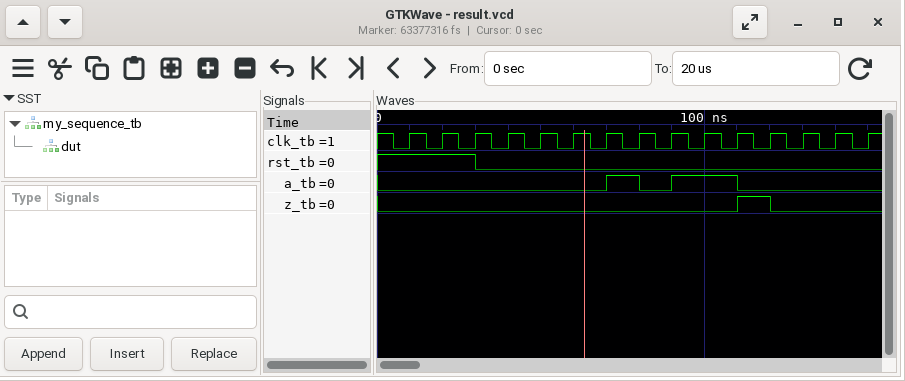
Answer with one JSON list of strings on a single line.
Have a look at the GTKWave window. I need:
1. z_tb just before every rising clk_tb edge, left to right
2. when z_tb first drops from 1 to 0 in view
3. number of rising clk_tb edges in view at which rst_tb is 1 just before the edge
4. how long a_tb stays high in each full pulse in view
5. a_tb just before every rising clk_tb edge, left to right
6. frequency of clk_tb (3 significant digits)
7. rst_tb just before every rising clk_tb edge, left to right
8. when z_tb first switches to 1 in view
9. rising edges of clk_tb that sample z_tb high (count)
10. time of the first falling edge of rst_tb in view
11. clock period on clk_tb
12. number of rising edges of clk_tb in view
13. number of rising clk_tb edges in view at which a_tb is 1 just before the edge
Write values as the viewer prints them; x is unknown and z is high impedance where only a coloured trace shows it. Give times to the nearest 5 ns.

["0 0 0 0 0 0 0 0 0 0 0 1 0 0 0", "120 ns", "3", "10 ns, 20 ns", "0 0 0 0 0 0 0 1 0 1 1 0 0 0 0", "100 MHz", "1 1 1 0 0 0 0 0 0 0 0 0 0 0 0", "110 ns", "1", "30 ns", "10 ns", "15", "3"]
